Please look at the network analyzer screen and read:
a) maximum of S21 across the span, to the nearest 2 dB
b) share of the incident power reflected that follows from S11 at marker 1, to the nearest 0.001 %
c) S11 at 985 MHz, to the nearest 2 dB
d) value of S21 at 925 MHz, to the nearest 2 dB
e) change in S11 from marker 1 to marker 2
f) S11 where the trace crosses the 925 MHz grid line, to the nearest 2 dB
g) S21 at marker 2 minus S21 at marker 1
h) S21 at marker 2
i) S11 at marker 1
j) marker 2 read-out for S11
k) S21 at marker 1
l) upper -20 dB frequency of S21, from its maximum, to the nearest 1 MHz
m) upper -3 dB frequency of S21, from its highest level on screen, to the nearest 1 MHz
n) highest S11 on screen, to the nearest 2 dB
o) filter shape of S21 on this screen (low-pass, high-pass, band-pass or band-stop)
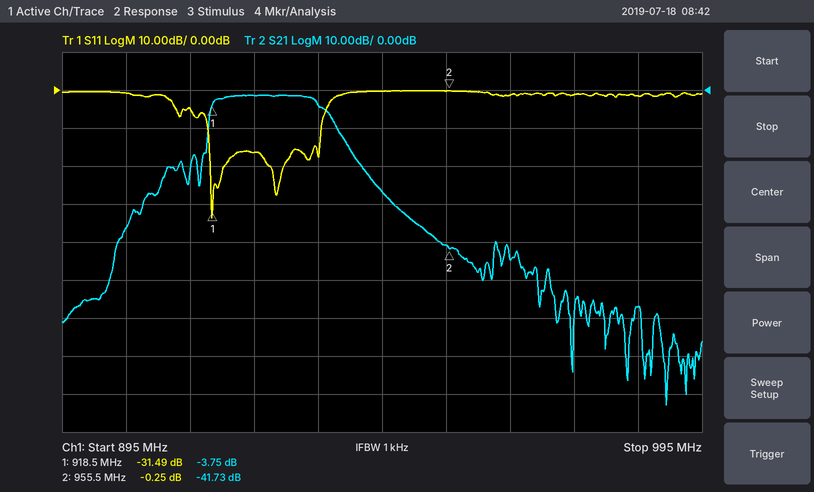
-2 dB
0.071 %
-2 dB
-2 dB
31.24 dB
-16 dB
-37.98 dB
-41.73 dB
-31.49 dB
-0.25 dB
-3.75 dB
942 MHz
935 MHz
0 dB
band-pass
